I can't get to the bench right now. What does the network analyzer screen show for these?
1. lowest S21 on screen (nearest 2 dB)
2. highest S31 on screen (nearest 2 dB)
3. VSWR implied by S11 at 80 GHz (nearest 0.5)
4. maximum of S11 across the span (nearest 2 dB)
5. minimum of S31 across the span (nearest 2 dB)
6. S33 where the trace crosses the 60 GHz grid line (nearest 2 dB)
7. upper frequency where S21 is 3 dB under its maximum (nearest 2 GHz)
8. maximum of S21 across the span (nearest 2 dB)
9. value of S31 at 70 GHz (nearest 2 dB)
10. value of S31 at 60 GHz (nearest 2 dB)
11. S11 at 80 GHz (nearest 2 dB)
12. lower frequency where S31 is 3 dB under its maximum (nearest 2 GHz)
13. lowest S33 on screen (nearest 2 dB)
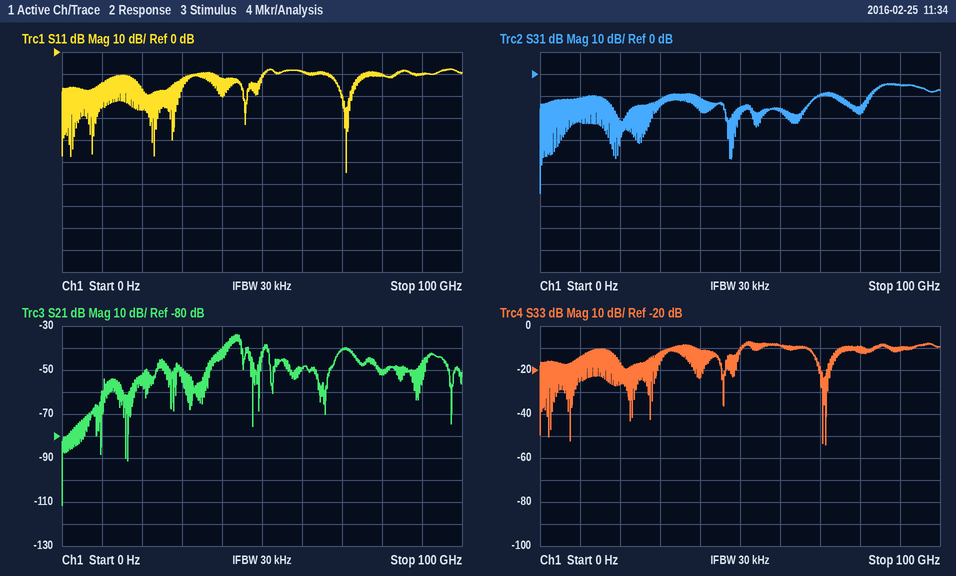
-112 dB
-4 dB
2.0
-8 dB
-54 dB
-8 dB
44 GHz
-34 dB
-10 dB
-16 dB
-10 dB
84 GHz
-54 dB
